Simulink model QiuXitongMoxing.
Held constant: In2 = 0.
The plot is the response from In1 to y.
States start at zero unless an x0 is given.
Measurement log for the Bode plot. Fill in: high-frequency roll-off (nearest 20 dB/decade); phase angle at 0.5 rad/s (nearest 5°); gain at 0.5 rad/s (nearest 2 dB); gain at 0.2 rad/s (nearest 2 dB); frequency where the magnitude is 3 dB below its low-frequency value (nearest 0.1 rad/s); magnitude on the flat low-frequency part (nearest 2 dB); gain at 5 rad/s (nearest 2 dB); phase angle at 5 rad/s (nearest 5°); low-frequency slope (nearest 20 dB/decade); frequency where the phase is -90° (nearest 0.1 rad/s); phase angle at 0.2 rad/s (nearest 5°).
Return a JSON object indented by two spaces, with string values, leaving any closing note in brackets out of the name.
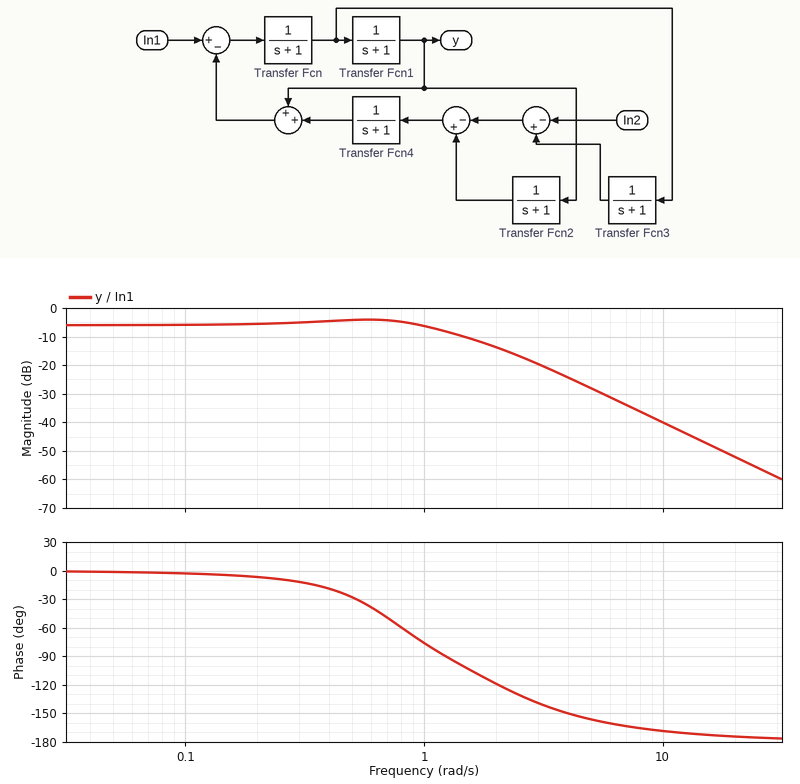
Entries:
{
  "high-frequency roll-off": "-40 dB/decade",
  "phase angle at 0.5 rad/s": "-30°",
  "gain at 0.5 rad/s": "-4 dB",
  "gain at 0.2 rad/s": "-6 dB",
  "frequency where the magnitude is 3 dB below its low-frequency value": "1.3 rad/s",
  "magnitude on the flat low-frequency part": "-6 dB",
  "gain at 5 rad/s": "-28 dB",
  "phase angle at 5 rad/s": "-155°",
  "low-frequency slope": "0 dB/decade",
  "frequency where the phase is -90°": "1.2 rad/s",
  "phase angle at 0.2 rad/s": "-5°"
}
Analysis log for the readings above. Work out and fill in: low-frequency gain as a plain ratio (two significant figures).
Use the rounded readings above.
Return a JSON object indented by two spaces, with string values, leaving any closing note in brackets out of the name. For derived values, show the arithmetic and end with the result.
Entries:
{
  "low-frequency gain as a plain ratio": "10^(-6 / 20) = 0.50"
}
